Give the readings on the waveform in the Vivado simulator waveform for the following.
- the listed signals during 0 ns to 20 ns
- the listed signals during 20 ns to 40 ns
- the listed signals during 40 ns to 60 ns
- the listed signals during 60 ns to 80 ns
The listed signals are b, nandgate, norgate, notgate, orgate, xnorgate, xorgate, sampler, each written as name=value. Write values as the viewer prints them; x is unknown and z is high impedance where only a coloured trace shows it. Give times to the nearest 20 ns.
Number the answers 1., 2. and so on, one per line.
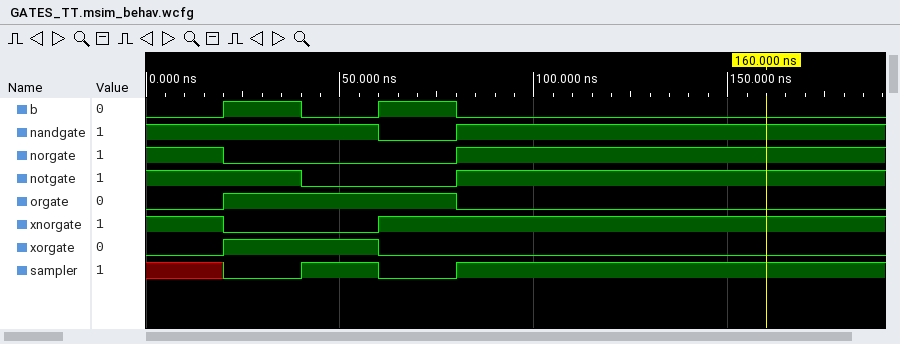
1. b=0, nandgate=1, norgate=1, notgate=1, orgate=0, xnorgate=1, xorgate=0, sampler=x
2. b=1, nandgate=1, norgate=0, notgate=1, orgate=1, xnorgate=0, xorgate=1, sampler=0
3. b=0, nandgate=1, norgate=0, notgate=0, orgate=1, xnorgate=0, xorgate=1, sampler=1
4. b=1, nandgate=0, norgate=0, notgate=0, orgate=1, xnorgate=1, xorgate=0, sampler=0
